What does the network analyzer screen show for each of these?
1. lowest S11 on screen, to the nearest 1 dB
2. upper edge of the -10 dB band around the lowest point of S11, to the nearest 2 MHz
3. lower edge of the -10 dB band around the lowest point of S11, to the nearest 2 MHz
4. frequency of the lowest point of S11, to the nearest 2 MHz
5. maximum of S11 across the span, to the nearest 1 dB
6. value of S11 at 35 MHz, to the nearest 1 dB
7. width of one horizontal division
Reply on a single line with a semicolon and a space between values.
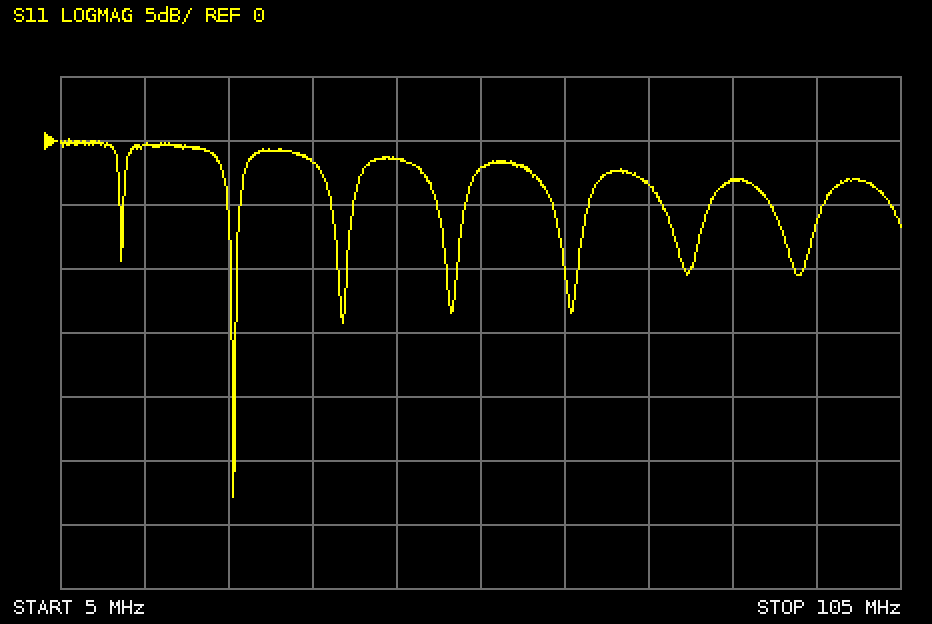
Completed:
-28 dB; 26 MHz; 26 MHz; 26 MHz; 0 dB; -2 dB; 10 MHz
